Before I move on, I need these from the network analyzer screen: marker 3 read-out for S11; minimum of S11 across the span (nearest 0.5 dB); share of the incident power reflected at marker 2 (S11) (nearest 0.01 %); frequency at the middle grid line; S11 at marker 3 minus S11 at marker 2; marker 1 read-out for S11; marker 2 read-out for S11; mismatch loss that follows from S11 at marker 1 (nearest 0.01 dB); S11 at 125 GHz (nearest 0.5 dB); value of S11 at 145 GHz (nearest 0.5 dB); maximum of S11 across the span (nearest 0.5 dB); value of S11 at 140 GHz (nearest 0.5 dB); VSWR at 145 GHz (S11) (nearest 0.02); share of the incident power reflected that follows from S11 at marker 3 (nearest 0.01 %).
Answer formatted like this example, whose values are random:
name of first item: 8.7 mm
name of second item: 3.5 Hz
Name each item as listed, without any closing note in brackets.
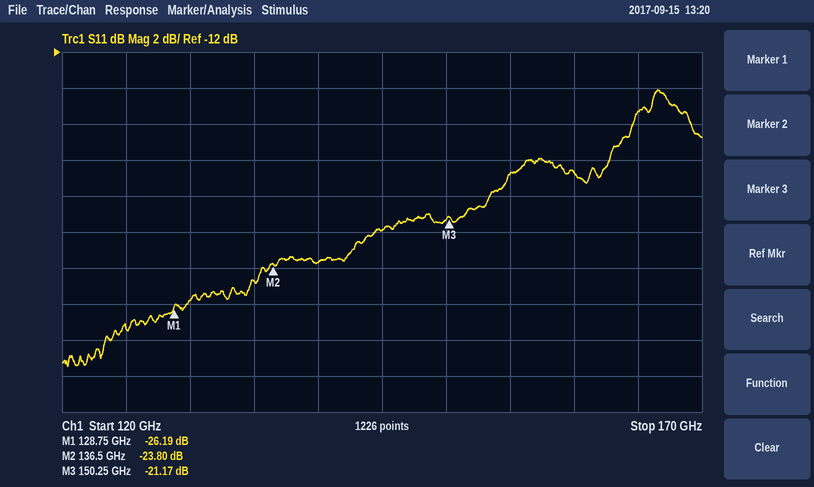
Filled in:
marker 3 read-out for S11: -21.17 dB
minimum of S11 across the span: -29.5 dB
share of the incident power reflected at marker 2 (S11): 0.42 %
frequency at the middle grid line: 145 GHz
S11 at marker 3 minus S11 at marker 2: 2.63 dB
marker 1 read-out for S11: -26.19 dB
marker 2 read-out for S11: -23.80 dB
mismatch loss that follows from S11 at marker 1: 0.01 dB
S11 at 125 GHz: -27.5 dB
value of S11 at 145 GHz: -22.0 dB
maximum of S11 across the span: -14.0 dB
value of S11 at 140 GHz: -23.5 dB
VSWR at 145 GHz (S11): 1.18
share of the incident power reflected that follows from S11 at marker 3: 0.76 %
